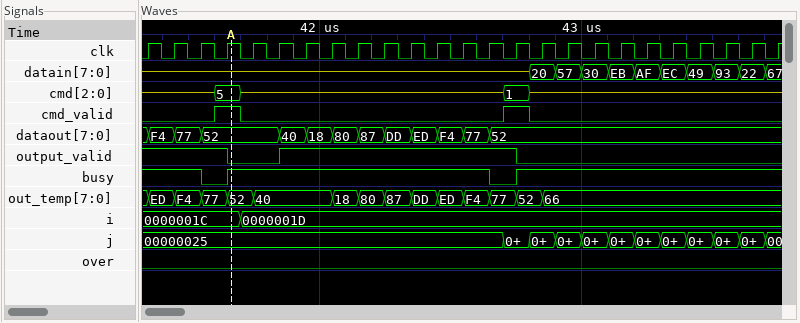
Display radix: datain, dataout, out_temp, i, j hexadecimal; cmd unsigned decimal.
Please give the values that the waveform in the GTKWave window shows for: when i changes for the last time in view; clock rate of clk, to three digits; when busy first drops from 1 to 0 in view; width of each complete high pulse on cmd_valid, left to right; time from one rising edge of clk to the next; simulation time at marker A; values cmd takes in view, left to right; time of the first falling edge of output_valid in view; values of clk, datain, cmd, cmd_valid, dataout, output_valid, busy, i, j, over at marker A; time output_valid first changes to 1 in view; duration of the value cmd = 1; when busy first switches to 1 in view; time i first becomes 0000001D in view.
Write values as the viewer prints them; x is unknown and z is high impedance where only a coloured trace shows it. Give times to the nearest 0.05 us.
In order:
41.7 us
10.0 MHz
41.55 us
0.1 us, 0.1 us
0.1 us
41.65 us
z, 5, z, 1, z
41.65 us
clk=1, datain=z, cmd=5, cmd_valid=1, dataout=52, output_valid=0, busy=1, i=0000001C, j=00000025, over=0
41.85 us
0.1 us
41.65 us
41.7 us
